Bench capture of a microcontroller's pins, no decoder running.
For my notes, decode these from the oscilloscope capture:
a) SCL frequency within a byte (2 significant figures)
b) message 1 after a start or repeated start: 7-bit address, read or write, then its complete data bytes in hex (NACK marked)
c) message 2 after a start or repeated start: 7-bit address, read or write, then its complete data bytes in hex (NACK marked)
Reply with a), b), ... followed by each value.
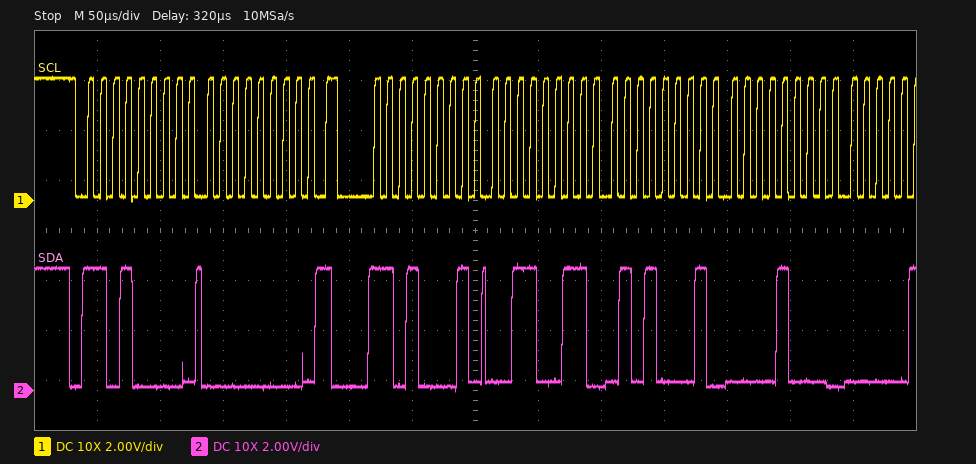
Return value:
a) 100 kHz
b) 0x68 write: 00
c) 0x68 read: 33 51 08
